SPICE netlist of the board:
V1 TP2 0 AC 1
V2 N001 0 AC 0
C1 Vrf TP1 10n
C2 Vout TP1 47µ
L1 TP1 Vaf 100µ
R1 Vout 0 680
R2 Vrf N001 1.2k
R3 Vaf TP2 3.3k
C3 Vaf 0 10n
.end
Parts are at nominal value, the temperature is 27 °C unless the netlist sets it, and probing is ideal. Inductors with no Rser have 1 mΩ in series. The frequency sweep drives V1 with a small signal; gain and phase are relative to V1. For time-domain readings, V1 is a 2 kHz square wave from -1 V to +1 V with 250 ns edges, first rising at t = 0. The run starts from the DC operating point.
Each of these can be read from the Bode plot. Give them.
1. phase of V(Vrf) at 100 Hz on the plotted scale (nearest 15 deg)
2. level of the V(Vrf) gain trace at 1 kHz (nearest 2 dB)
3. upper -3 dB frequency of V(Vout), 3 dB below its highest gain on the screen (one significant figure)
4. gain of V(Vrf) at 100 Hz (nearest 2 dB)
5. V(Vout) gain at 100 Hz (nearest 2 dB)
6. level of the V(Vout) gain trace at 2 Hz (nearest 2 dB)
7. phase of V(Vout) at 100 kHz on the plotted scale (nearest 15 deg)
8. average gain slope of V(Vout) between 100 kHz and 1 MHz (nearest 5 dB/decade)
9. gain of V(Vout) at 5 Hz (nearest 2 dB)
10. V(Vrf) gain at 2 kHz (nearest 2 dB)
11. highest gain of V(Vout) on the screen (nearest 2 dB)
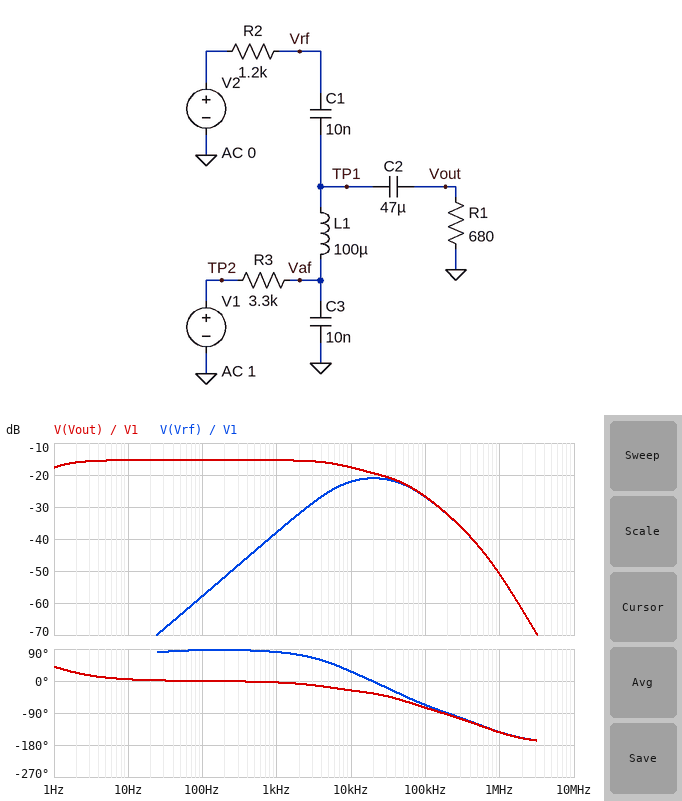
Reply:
90 deg
-38 dB
10 kHz
-58 dB
-16 dB
-16 dB
-75 deg
-25 dB/decade
-16 dB
-32 dB
-16 dB
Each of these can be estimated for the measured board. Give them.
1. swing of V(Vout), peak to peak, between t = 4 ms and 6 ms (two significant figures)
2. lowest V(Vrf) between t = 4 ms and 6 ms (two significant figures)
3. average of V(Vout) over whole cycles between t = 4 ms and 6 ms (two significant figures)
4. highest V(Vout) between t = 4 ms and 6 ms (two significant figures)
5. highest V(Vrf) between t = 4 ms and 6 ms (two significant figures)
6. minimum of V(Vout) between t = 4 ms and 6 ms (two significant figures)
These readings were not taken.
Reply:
340 mV
-150 mV
170 mV
340 mV
150 mV
-5.4 mV
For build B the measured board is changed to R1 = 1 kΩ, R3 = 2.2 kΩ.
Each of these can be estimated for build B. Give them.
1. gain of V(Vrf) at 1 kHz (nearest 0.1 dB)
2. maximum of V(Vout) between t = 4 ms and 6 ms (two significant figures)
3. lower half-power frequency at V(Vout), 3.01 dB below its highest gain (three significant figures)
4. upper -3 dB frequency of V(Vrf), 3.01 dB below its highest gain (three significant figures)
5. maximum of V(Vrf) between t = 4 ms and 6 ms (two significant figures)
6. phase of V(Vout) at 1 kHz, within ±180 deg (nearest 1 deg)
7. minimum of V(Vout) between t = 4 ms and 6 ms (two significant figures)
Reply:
-32.6 dB
620 mV
1.06 Hz
57.0 kHz
240 mV
-5 deg
-12 mV
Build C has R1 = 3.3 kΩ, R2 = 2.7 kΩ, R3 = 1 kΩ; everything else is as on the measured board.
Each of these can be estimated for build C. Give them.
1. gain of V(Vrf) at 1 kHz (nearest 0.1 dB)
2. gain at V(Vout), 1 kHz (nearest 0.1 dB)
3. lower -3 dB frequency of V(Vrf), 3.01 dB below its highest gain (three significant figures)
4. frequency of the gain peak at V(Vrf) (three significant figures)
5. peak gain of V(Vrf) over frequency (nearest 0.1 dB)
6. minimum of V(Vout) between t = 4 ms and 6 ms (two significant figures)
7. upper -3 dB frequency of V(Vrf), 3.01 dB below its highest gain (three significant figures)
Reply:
-17.9 dB
-2.4 dB
3.41 kHz
11.1 kHz
-6.2 dB
-22 mV
36.1 kHz
